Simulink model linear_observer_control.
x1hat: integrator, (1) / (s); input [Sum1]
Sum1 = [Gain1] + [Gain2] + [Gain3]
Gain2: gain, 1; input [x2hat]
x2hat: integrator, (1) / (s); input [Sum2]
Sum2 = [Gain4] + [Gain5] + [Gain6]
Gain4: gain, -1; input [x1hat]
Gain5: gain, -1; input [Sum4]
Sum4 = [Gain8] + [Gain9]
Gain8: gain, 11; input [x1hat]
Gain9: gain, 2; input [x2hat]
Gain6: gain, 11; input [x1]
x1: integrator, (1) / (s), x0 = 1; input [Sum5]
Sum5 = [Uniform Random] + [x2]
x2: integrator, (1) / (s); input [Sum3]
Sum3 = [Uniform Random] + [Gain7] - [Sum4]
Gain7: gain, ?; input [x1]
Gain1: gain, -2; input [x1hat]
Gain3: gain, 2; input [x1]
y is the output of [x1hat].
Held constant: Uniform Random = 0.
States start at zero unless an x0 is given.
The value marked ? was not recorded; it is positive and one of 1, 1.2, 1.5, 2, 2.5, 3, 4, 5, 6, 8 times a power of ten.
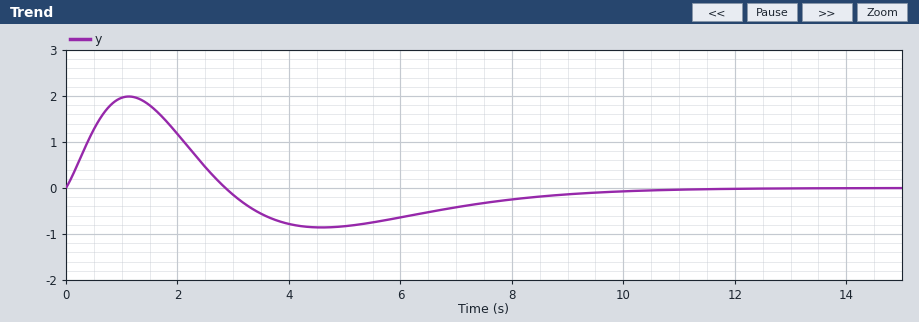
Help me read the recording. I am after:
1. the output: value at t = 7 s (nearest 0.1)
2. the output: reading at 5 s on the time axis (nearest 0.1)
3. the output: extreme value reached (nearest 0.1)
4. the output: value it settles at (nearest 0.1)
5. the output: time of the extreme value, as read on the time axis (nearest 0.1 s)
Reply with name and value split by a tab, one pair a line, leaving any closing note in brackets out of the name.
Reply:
the output: value at t = 7 s	-0.4
the output: reading at 5 s on the time axis	-0.8
the output: extreme value reached	2.0
the output: value it settles at	0.0
the output: time of the extreme value, as read on the time axis	1.1 s
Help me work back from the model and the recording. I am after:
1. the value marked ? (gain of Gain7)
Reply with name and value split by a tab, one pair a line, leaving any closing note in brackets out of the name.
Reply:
the value marked ?	10
